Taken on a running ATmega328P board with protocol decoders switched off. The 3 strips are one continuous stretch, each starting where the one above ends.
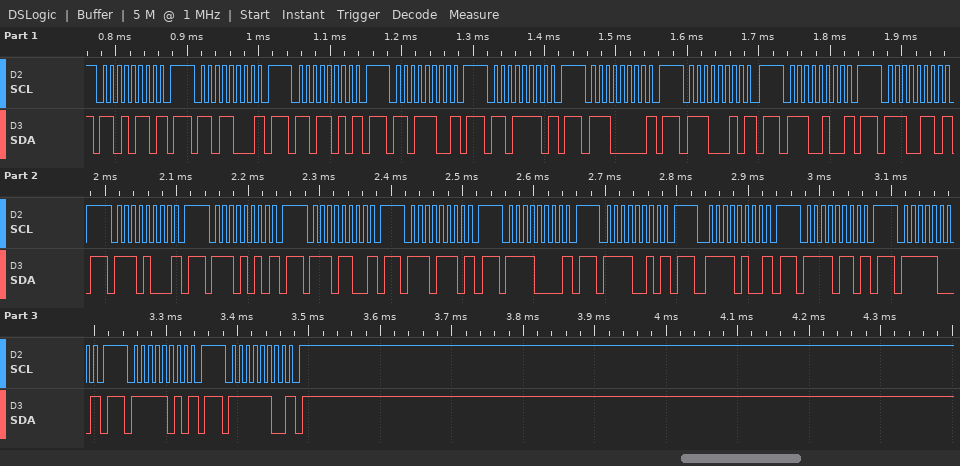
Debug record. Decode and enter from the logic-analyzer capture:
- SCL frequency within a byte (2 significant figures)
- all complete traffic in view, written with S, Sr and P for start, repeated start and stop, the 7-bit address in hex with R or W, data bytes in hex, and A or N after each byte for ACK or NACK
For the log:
100 kHz
S 6BW N P S 6CW N P S 6DW N P S 6EW N P S 6FW N P S 70W N P S 71W N P S 72W N P S 73W N P S 74W N P S 75W N P S 76W N P S 77W N P S 78W N P S 79W N P S 7AW N P S 7BW N P S 7CW N P S 7DW N P S 7EW N P
